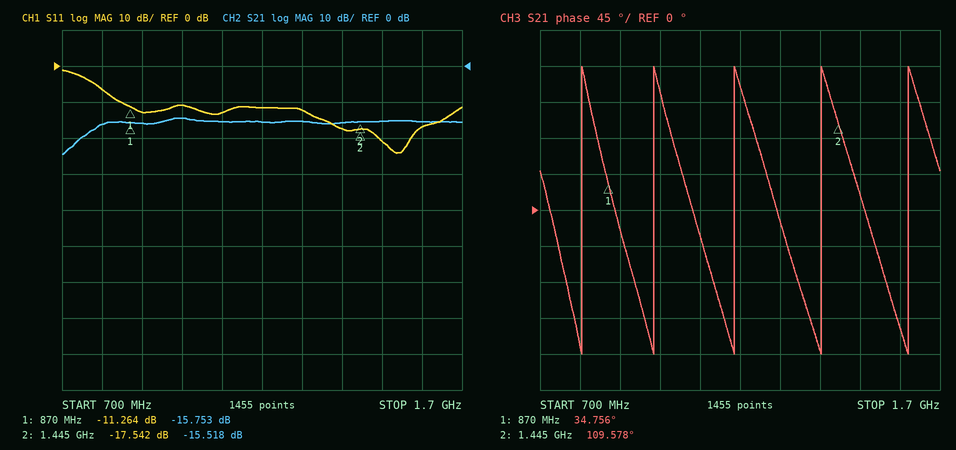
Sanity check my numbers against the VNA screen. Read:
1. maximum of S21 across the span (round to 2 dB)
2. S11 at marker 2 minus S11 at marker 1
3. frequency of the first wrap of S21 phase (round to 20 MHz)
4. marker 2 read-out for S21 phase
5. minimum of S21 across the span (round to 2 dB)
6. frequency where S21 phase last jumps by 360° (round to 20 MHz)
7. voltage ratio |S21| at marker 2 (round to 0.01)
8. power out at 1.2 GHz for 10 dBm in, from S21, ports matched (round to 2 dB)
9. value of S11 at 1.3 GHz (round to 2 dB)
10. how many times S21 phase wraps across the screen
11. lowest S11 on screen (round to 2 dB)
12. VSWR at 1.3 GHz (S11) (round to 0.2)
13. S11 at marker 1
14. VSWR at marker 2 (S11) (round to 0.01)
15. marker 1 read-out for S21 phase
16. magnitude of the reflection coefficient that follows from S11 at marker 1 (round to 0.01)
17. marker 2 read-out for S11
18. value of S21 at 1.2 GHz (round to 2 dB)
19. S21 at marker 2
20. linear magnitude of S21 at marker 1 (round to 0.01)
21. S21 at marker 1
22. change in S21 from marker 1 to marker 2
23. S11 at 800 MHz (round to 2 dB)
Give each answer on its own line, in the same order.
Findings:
-14 dB
-6.278 dB
800 MHz
109.578°
-24 dB
1.62 GHz
0.17
-6 dBm
-12 dB
5
-24 dB
1.6
-11.264 dB
1.31
34.756°
0.27
-17.542 dB
-16 dB
-15.518 dB
0.16
-15.753 dB
0.235 dB
-6 dB
